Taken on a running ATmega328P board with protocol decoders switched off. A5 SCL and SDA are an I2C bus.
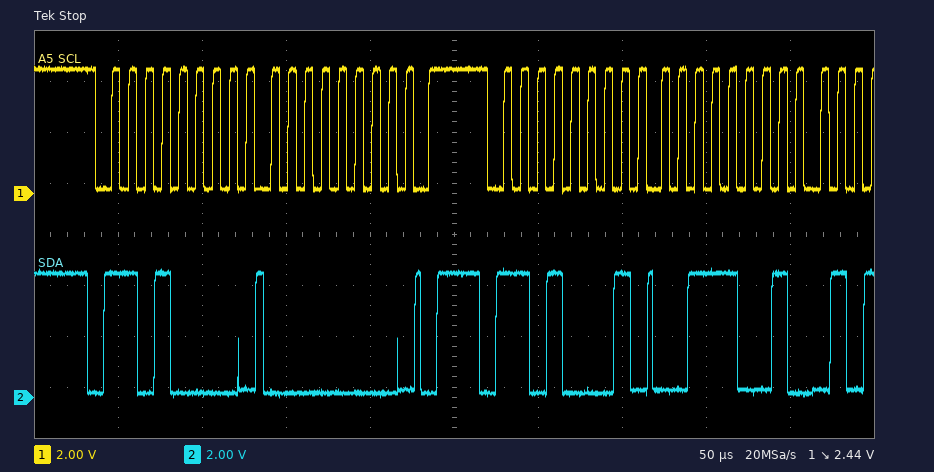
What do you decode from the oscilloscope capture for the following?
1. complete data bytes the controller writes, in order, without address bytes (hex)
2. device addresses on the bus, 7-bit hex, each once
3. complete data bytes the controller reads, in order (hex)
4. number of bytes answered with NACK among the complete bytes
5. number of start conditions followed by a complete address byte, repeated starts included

00
0x68
39
0
2
